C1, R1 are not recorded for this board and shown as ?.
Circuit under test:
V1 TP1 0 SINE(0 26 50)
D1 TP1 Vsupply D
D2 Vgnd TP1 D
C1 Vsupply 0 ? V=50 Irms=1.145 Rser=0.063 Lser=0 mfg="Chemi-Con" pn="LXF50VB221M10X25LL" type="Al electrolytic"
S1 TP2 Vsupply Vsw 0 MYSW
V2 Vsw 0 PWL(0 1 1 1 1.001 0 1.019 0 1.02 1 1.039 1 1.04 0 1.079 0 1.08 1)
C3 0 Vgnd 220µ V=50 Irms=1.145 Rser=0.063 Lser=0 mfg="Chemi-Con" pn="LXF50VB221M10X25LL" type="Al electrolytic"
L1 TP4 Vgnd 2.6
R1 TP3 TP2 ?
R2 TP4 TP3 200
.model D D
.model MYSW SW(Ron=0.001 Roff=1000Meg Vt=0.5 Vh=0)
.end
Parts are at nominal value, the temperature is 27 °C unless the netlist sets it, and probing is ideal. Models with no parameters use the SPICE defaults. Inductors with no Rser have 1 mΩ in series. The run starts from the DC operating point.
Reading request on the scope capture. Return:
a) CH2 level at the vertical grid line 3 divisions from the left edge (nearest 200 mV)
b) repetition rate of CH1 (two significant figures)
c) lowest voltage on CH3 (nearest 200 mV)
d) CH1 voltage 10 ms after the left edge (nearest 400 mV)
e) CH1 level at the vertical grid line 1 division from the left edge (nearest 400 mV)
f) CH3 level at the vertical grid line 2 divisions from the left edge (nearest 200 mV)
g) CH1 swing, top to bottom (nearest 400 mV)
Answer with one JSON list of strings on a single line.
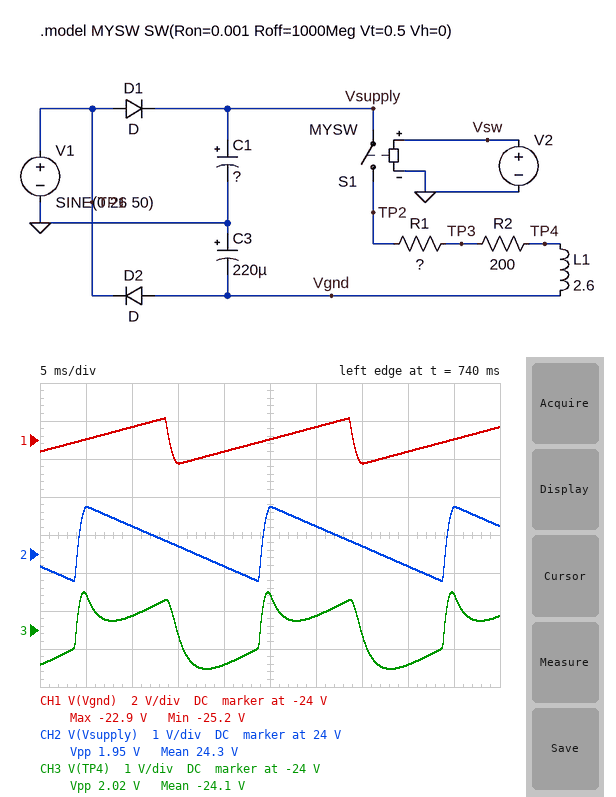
["24.2 V", "50 Hz", "-25.0 V", "-23.2 V", "-24.0 V", "-23.6 V", "2.4 V"]
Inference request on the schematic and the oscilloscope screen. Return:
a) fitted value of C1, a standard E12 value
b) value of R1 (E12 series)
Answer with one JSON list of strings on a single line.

["270 µF", "1.5 kΩ"]
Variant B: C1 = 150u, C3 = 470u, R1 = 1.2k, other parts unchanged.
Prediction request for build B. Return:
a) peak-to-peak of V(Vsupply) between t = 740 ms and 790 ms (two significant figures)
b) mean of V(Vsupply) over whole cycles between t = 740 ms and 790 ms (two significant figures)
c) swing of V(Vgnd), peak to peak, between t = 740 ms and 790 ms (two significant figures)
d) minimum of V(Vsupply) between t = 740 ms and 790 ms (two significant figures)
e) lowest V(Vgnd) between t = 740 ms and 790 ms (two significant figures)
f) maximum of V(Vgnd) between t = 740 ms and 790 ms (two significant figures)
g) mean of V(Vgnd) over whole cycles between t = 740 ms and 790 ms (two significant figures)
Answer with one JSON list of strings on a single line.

["4.1 V", "23 V", "1.4 V", "21 V", "-25 V", "-24 V", "-25 V"]
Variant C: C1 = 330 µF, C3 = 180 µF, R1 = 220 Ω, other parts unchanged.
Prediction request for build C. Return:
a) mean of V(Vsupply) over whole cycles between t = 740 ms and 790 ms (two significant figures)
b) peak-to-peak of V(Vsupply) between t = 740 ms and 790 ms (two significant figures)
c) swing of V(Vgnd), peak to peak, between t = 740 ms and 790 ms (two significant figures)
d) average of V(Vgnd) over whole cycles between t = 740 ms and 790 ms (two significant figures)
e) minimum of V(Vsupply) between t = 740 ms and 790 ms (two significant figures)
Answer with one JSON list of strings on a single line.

["23 V", "5.5 V", "9.7 V", "-21 V", "20 V"]
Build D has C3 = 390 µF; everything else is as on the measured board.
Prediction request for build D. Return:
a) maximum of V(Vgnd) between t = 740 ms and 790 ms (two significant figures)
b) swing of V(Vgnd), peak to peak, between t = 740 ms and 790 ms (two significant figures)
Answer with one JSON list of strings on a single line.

["-24 V", "1.4 V"]
